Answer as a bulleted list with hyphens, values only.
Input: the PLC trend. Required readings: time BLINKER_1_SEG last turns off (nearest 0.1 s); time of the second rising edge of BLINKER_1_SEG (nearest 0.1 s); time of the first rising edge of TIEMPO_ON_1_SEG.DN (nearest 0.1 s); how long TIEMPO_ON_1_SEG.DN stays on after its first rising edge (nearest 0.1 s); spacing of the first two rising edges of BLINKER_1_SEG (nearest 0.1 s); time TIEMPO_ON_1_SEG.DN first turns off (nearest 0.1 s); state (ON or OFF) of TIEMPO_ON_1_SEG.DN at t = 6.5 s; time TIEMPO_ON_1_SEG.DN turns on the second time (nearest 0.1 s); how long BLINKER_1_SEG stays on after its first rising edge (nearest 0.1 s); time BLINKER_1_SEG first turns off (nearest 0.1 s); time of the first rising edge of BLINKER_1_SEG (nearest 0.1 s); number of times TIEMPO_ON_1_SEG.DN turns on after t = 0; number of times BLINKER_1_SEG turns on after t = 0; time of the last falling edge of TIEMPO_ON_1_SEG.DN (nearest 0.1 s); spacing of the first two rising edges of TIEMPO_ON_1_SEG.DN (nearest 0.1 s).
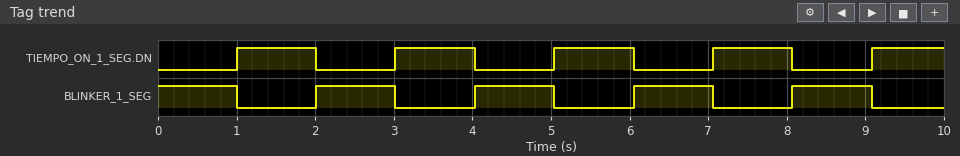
- 9.1 s
- 4.0 s
- 1.0 s
- 1.0 s
- 2.0 s
- 2.0 s
- OFF
- 3.0 s
- 1.0 s
- 1.0 s
- 2.0 s
- 5
- 4
- 8.1 s
- 2.0 s
